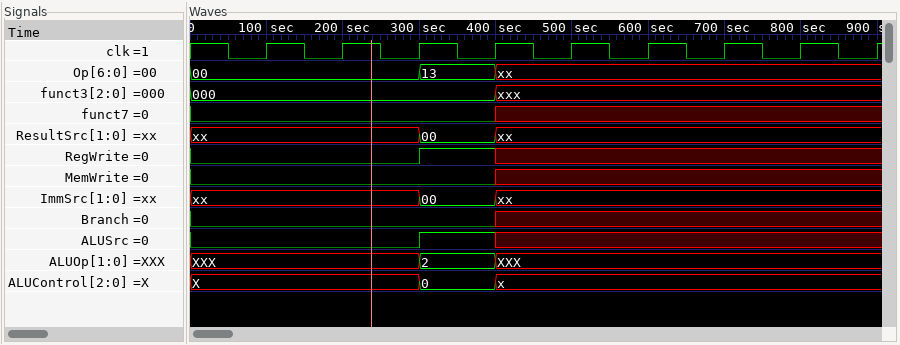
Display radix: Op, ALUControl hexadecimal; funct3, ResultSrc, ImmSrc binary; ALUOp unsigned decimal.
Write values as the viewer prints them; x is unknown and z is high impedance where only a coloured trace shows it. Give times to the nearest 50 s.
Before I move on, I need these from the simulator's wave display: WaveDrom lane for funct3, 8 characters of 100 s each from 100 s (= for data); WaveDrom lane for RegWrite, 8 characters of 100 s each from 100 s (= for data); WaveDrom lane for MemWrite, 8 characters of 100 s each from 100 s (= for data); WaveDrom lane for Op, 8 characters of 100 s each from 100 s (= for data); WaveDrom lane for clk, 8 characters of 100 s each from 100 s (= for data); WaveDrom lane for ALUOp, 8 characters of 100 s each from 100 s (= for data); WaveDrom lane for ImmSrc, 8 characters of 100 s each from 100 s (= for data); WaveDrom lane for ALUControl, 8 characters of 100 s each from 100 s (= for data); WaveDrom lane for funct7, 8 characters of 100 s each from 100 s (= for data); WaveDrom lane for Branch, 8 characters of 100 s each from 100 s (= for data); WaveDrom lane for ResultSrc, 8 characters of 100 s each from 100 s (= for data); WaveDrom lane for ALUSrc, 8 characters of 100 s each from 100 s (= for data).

{name: 'funct3', wave: '=..x....', data: '000'}
{name: 'RegWrite', wave: '0.1x....'}
{name: 'MemWrite', wave: '0..x....'}
{name: 'Op', wave: '=.=x....', data: '00 13'}
{name: 'clk', wave: 'p.......'}
{name: 'ALUOp', wave: 'x.=x....', data: '2'}
{name: 'ImmSrc', wave: 'x.=x....', data: '00'}
{name: 'ALUControl', wave: '=.=x....', data: 'X 0'}
{name: 'funct7', wave: '0..x....'}
{name: 'Branch', wave: '0..x....'}
{name: 'ResultSrc', wave: 'x.=x....', data: '00'}
{name: 'ALUSrc', wave: '0.1x....'}
